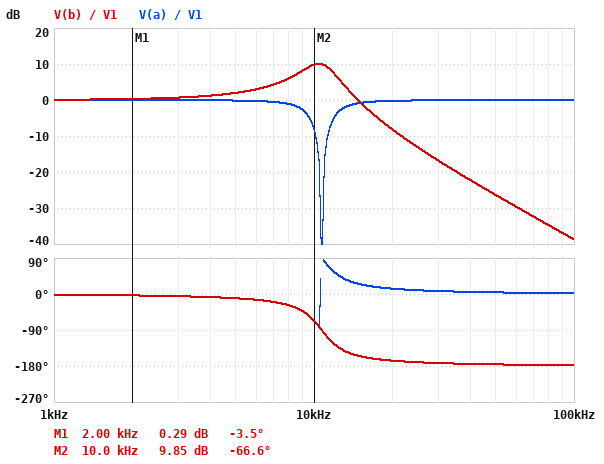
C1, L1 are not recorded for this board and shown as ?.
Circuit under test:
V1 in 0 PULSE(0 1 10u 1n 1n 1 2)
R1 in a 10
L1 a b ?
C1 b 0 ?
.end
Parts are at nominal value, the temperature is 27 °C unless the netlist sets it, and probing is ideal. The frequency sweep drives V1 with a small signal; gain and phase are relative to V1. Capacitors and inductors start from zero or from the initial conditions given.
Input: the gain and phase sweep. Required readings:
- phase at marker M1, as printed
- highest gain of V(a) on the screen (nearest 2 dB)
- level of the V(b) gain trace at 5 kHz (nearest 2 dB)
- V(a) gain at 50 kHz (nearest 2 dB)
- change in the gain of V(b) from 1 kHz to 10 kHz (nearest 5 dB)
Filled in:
-3.5 deg
0 dB
2 dB
0 dB
10 dB
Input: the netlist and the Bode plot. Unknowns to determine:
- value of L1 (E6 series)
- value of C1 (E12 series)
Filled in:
470 µH
470 nF
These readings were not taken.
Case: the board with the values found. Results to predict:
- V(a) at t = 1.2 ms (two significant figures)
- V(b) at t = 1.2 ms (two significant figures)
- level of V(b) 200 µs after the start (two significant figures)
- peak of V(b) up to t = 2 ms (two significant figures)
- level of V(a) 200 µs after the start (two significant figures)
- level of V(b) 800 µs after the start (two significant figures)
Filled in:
1.0 V
1.0 V
870 mV
1.6 V
1.0 V
1.0 V
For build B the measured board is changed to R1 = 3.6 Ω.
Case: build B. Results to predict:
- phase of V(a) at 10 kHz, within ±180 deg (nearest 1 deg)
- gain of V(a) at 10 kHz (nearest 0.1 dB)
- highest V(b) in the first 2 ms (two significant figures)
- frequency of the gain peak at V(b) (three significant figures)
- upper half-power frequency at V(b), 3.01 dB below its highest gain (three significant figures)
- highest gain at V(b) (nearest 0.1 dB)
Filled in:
-40 deg
-2.3 dB
1.8 V
10.7 kHz
11.3 kHz
18.9 dB
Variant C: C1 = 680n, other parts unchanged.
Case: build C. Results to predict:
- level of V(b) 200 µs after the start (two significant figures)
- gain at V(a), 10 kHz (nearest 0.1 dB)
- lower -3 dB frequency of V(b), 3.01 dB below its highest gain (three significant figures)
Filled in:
1.1 V
-5.6 dB
6.63 kHz
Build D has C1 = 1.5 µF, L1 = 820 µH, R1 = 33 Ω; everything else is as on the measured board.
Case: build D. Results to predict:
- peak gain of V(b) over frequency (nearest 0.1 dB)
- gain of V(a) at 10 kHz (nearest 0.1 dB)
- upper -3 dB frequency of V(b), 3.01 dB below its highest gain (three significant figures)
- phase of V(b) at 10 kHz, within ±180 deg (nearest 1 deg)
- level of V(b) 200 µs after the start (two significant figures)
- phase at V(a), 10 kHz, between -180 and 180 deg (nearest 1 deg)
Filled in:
0 dB
-2.2 dB
4.55 kHz
-141 deg
1.0 V
39 deg
